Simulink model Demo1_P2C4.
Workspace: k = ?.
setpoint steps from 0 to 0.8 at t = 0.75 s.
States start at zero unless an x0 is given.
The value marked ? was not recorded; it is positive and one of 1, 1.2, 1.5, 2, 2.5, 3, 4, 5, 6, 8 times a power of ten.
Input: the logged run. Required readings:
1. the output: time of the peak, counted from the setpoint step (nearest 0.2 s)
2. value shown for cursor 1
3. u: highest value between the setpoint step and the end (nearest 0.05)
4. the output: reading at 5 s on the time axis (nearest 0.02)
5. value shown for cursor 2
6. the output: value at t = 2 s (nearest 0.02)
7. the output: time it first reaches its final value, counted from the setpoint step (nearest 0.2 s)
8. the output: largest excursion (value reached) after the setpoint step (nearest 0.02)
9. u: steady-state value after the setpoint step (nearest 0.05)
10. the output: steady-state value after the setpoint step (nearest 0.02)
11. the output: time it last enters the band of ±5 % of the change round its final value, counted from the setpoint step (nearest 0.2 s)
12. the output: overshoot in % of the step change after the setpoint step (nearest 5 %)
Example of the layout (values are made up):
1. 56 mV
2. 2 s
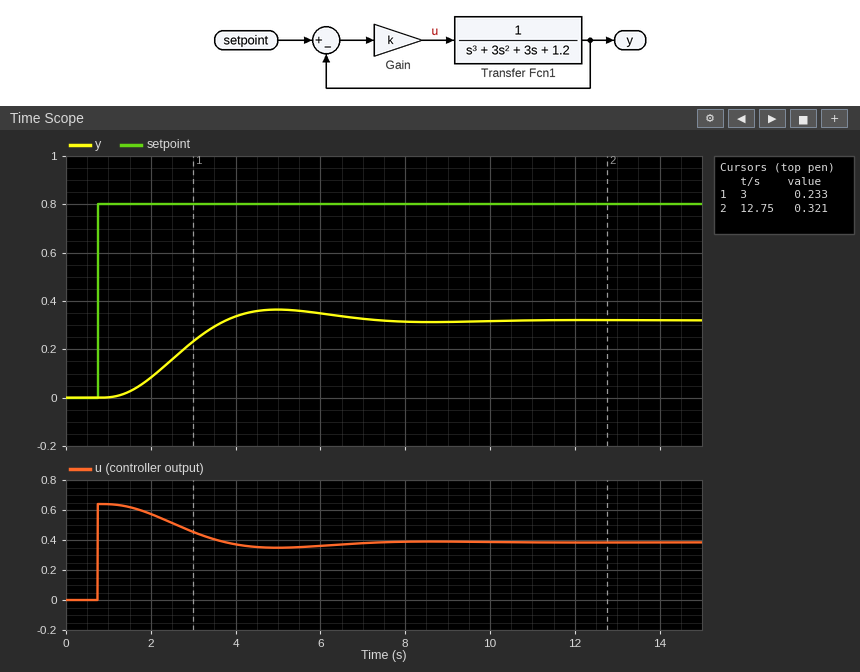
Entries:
1. 4.2 s
2. 0.233
3. 0.65
4. 0.36
5. 0.321
6. 0.08
7. 3.0 s
8. 0.36
9. 0.40
10. 0.32
11. 5.8 s
12. 15 %
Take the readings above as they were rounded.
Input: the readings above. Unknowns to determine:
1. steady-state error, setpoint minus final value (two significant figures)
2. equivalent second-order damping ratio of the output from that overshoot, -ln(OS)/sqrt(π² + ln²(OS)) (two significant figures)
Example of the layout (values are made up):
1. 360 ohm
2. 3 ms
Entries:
1. 0.48
2. 0.52
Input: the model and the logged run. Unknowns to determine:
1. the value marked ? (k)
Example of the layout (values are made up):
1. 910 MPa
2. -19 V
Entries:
1. 0.8
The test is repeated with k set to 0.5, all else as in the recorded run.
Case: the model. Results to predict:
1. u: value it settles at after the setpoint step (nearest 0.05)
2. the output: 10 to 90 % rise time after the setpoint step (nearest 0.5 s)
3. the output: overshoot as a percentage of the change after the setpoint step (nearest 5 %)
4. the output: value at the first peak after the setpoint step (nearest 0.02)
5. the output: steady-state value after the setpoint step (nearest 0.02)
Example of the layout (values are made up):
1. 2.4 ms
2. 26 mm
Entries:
1. 0.30
2. 2.0 s
3. 10 %
4. 0.26
5. 0.24
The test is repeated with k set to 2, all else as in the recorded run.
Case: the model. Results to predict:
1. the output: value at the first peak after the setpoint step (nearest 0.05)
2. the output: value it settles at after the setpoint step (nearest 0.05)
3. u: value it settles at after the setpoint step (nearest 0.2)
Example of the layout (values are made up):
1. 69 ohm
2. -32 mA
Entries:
1. 0.65
2. 0.50
3. 0.6
